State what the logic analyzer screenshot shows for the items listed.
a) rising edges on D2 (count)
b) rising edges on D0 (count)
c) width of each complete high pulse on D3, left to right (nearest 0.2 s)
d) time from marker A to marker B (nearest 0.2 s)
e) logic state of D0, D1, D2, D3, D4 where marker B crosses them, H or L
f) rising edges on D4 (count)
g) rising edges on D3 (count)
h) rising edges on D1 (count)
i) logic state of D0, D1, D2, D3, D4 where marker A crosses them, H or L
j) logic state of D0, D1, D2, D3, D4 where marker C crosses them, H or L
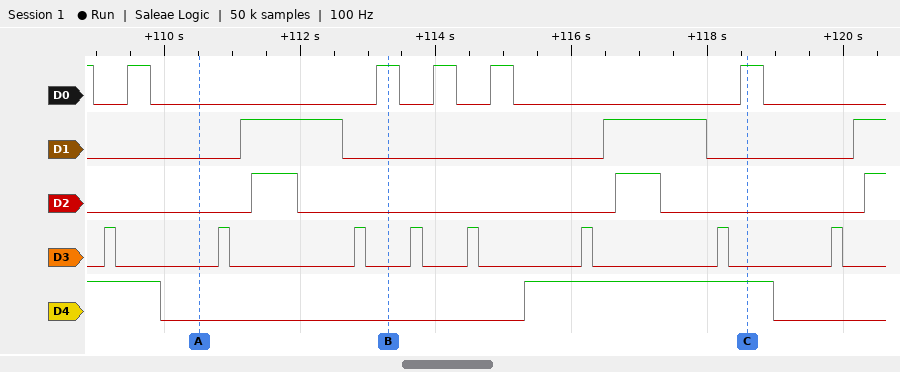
3
5
0.2 s, 0.2 s, 0.2 s, 0.2 s, 0.2 s, 0.2 s, 0.2 s, 0.2 s
2.8 s
D0=H, D1=L, D2=L, D3=L, D4=L
1
8
3
D0=L, D1=L, D2=L, D3=L, D4=L
D0=H, D1=L, D2=L, D3=L, D4=H
